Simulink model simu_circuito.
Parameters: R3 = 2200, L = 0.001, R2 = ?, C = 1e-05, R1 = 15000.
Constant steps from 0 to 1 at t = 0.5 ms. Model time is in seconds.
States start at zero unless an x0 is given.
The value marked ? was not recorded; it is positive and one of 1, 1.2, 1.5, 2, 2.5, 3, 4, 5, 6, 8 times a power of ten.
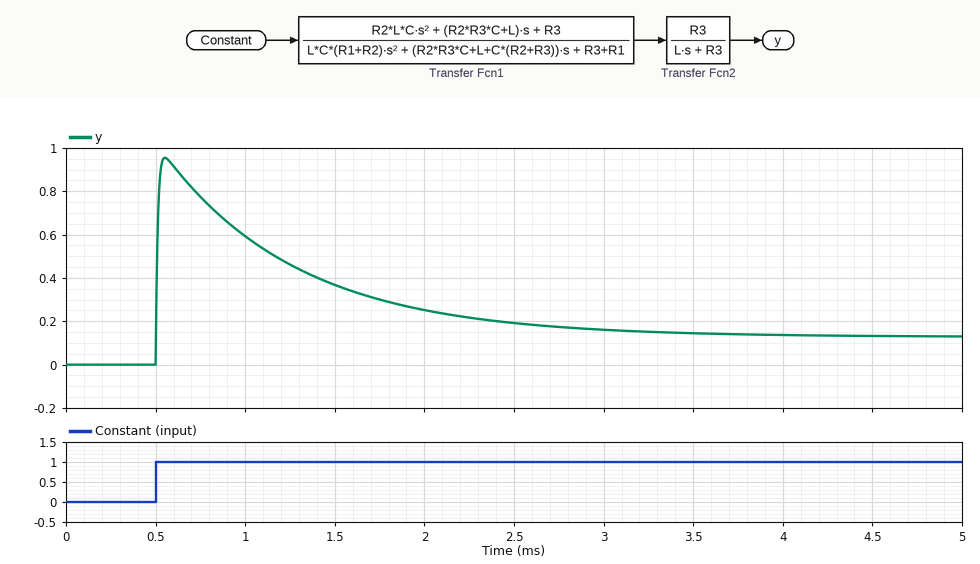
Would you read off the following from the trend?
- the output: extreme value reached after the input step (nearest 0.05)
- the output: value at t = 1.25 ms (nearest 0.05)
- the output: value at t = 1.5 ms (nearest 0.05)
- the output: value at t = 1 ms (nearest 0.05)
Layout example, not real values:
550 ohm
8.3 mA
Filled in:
0.95
0.45
0.35
0.60
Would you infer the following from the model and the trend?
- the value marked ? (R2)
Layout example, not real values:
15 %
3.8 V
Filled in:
600
